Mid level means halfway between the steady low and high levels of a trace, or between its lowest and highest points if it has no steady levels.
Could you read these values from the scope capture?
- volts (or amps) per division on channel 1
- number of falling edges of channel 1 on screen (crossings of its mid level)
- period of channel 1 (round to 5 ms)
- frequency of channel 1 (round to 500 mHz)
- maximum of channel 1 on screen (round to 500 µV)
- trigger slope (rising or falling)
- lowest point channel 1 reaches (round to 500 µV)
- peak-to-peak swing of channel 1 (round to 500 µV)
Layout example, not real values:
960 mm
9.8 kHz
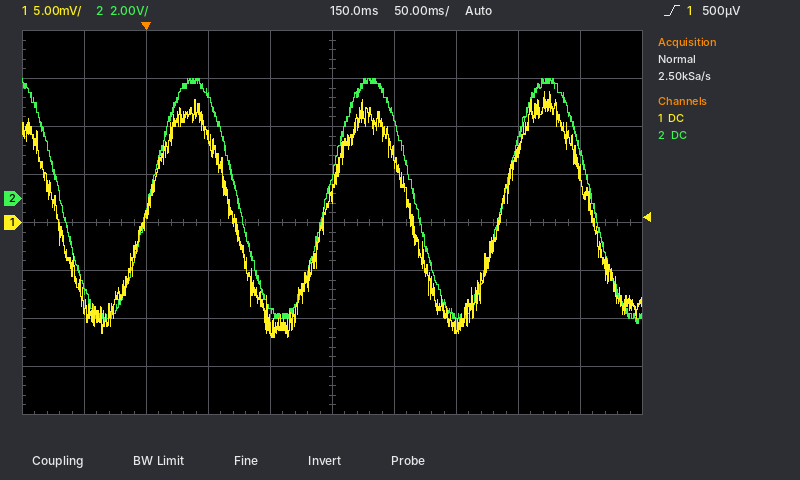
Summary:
5 mV
4
145 ms
7.0 Hz
13.5 mV
rising
-12.0 mV
25.5 mV
